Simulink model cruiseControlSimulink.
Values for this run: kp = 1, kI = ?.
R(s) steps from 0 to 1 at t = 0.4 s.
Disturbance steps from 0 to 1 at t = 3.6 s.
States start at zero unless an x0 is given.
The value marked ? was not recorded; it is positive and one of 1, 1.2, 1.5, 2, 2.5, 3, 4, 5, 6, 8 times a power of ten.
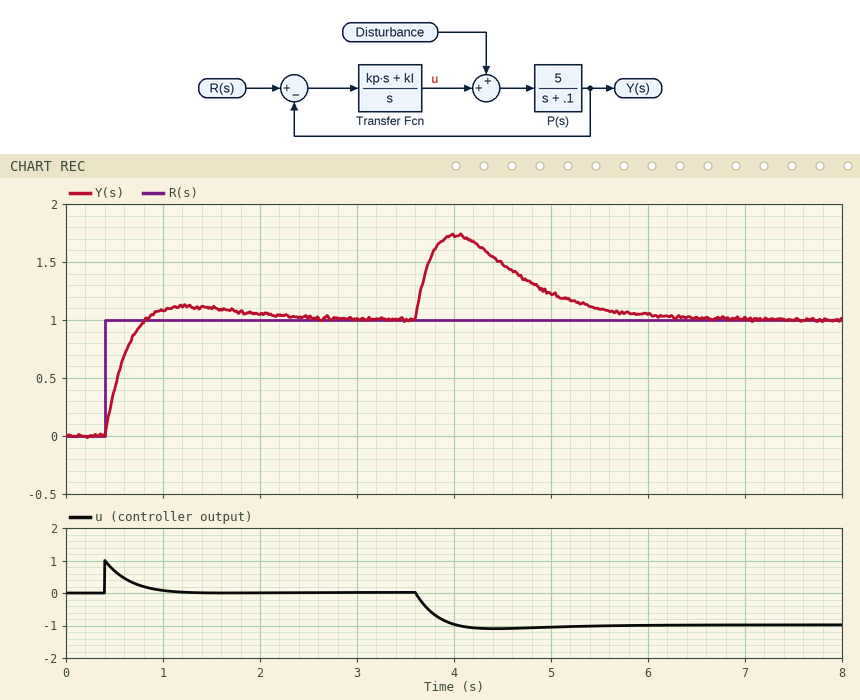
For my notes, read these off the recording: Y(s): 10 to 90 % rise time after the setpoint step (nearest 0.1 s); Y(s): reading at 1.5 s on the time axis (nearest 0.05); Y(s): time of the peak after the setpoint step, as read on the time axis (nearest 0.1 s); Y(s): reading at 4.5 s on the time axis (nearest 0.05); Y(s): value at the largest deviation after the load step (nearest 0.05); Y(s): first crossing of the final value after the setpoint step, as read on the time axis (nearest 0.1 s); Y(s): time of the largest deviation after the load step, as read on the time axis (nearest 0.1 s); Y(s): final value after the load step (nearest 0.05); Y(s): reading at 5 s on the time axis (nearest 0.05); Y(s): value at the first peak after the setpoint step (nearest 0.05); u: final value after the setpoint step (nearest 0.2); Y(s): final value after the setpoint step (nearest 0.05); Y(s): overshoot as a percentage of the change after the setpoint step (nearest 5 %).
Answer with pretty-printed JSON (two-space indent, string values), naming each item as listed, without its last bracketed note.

{
  "Y(s): 10 to 90 % rise time after the setpoint step": "0.3 s",
  "Y(s): reading at 1.5 s on the time axis": "1.10",
  "Y(s): time of the peak after the setpoint step, as read on the time axis": "1.2 s",
  "Y(s): reading at 4.5 s on the time axis": "1.50",
  "Y(s): value at the largest deviation after the load step": "1.75",
  "Y(s): first crossing of the final value after the setpoint step, as read on the time axis": "0.8 s",
  "Y(s): time of the largest deviation after the load step, as read on the time axis": "4.0 s",
  "Y(s): final value after the load step": "1.00",
  "Y(s): reading at 5 s on the time axis": "1.25",
  "Y(s): value at the first peak after the setpoint step": "1.10",
  "u: final value after the setpoint step": "0.0",
  "Y(s): final value after the setpoint step": "1.00",
  "Y(s): overshoot as a percentage of the change after the setpoint step": "10 %"
}
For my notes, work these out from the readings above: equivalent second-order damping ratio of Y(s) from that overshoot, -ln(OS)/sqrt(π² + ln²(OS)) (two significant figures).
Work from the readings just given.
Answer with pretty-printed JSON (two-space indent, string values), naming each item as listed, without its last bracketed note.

{
  "equivalent second-order damping ratio of Y(s) from that overshoot, -ln(OS)/sqrt(π² + ln²(OS))": "0.59"
}
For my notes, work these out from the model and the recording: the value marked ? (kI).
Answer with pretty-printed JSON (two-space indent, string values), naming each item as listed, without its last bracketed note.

{
  "the value marked ?": "1.2"
}
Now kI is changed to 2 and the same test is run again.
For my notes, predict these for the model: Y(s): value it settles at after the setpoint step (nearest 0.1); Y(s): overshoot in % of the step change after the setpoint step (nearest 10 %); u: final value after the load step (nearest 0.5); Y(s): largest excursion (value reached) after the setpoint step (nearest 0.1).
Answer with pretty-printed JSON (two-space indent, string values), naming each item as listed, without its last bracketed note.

{
  "Y(s): value it settles at after the setpoint step": "1.0",
  "Y(s): overshoot in % of the step change after the setpoint step": "20 %",
  "u: final value after the load step": "-1.0",
  "Y(s): largest excursion (value reached) after the setpoint step": "1.2"
}
